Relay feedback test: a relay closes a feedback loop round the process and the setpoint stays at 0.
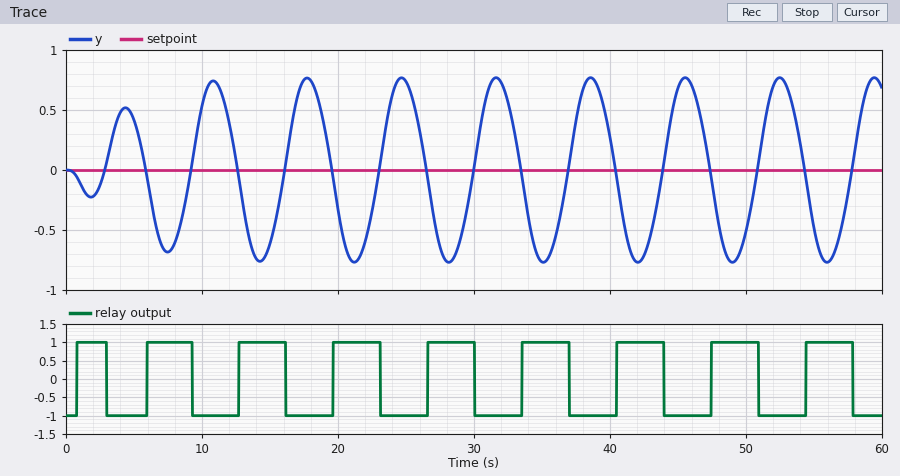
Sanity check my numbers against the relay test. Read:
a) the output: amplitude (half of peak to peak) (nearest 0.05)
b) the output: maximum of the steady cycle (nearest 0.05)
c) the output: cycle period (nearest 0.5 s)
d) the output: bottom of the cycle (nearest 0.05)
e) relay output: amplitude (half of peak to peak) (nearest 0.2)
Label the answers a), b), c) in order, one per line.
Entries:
a) 0.75
b) 0.75
c) 7.0 s
d) -0.75
e) 1.0
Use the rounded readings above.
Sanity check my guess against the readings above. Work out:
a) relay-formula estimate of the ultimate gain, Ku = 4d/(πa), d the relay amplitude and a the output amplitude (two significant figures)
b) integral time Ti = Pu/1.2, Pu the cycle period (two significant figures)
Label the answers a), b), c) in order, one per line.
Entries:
a) 1.7
b) 5.8 s
